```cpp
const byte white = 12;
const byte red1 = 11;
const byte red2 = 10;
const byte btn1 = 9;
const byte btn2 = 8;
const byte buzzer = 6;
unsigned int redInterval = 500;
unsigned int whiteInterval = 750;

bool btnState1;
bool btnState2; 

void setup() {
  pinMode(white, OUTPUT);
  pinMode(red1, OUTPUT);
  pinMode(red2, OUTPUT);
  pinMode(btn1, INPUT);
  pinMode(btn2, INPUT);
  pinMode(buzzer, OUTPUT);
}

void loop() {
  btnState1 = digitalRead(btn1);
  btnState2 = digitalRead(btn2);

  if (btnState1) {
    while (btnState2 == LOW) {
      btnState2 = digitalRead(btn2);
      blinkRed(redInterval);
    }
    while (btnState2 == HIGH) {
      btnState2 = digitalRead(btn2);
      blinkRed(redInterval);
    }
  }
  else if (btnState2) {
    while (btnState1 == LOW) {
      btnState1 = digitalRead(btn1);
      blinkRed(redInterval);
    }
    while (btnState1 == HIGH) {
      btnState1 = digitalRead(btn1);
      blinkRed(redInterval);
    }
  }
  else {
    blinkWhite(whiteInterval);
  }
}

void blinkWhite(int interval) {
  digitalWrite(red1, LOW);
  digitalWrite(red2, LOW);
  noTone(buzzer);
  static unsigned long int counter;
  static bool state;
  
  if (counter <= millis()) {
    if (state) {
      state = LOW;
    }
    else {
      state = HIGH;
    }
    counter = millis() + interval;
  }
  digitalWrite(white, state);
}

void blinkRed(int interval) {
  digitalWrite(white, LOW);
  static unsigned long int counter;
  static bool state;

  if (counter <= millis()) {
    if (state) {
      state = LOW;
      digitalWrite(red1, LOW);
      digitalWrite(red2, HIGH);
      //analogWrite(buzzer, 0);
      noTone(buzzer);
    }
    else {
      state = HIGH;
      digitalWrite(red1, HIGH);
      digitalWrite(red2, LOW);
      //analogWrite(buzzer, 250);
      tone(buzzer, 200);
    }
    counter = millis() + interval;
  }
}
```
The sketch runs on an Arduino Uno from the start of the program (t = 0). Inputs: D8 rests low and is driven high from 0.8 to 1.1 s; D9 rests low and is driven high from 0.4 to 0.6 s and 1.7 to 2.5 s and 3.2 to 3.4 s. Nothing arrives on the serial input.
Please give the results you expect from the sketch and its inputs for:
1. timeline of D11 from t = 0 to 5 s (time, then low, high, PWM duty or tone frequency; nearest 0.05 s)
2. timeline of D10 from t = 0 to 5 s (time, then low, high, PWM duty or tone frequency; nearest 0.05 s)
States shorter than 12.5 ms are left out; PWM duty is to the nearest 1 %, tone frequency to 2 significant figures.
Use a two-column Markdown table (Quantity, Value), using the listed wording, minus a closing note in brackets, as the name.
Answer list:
| Quantity | Value |
|---|---|
| timeline of D11 from t = 0 to 5 s | 0 s low; 0.4 s high; 0.9 s low; 1.7 s high; 2.2 s low; 2.7 s high; 3.2 s low; 3.7 s high; 4.2 s low; 4.7 s high |
| timeline of D10 from t = 0 to 5 s | 0 s low; 0.9 s high; 1.1 s low; 2.2 s high; 2.7 s low; 3.2 s high; 3.7 s low; 4.2 s high; 4.7 s low |
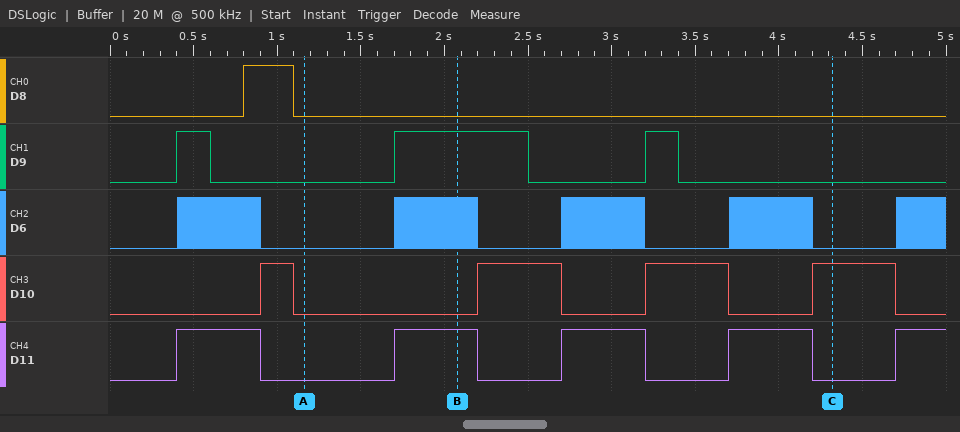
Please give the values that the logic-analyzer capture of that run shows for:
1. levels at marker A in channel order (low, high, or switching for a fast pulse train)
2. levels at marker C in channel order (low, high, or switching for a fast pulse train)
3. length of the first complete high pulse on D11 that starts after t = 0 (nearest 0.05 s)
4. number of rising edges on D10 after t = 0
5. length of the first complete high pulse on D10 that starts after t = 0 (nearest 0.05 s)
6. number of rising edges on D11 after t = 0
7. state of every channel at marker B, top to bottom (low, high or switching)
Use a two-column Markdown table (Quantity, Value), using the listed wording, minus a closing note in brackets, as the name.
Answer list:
| Quantity | Value |
|---|---|
| levels at marker A in channel order | D8 low, D9 low, D6 low, D10 low, D11 low |
| levels at marker C in channel order | D8 low, D9 low, D6 low, D10 high, D11 low |
| length of the first complete high pulse on D11 that starts after t = 0 | 0.50 s |
| number of rising edges on D10 after t = 0 | 4 |
| length of the first complete high pulse on D10 that starts after t = 0 | 0.20 s |
| number of rising edges on D11 after t = 0 | 5 |
| state of every channel at marker B, top to bottom | D8 low, D9 high, D6 switching, D10 low, D11 high |
